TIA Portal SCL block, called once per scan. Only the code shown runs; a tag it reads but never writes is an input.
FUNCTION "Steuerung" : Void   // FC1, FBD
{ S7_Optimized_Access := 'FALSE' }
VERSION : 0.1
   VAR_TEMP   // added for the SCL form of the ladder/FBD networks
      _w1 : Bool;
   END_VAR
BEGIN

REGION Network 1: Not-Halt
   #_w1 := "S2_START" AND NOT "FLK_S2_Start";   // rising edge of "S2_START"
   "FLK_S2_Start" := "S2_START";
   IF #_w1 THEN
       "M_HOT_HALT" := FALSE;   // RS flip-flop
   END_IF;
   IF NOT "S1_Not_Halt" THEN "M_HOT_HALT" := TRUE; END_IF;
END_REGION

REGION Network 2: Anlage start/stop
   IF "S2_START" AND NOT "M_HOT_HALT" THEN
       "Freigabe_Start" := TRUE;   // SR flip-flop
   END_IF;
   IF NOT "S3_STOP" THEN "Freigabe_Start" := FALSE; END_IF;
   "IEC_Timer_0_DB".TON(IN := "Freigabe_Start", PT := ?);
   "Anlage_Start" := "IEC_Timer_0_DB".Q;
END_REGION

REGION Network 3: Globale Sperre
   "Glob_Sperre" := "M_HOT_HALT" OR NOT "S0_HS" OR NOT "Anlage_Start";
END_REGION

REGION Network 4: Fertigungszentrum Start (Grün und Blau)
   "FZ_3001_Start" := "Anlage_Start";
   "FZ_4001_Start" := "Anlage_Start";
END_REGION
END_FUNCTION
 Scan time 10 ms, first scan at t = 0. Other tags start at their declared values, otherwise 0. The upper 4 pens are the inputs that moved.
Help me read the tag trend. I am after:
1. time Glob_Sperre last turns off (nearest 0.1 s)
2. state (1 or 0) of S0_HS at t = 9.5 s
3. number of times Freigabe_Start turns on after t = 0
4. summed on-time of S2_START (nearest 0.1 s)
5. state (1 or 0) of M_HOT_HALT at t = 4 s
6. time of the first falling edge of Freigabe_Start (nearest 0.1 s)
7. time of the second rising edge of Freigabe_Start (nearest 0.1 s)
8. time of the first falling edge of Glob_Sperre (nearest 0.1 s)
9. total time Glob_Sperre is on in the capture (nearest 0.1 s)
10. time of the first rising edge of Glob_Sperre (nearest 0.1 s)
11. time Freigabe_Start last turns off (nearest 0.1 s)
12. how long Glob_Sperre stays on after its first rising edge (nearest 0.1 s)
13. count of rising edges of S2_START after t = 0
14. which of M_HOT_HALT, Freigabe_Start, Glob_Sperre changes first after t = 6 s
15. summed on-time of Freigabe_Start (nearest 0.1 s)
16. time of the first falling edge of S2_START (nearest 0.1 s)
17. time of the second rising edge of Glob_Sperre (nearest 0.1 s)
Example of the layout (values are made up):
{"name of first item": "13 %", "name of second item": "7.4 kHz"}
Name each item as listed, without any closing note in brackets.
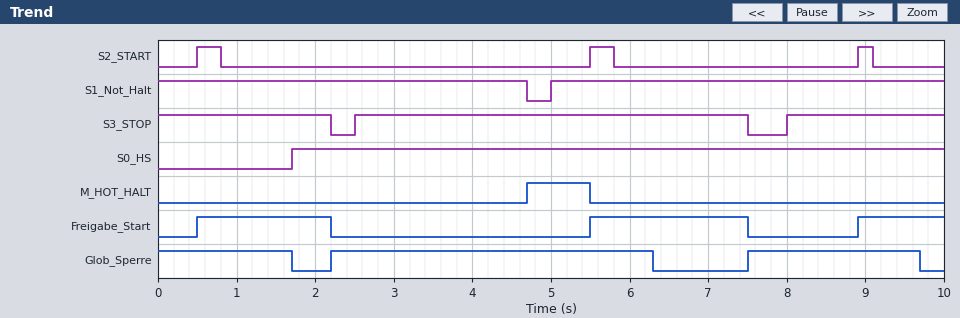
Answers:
{"time Glob_Sperre last turns off": "9.7 s", "state (1 or 0) of S0_HS at t = 9.5 s": "1", "number of times Freigabe_Start turns on after t = 0": "3", "summed on-time of S2_START": "0.8 s", "state (1 or 0) of M_HOT_HALT at t = 4 s": "0", "time of the first falling edge of Freigabe_Start": "2.2 s", "time of the second rising edge of Freigabe_Start": "5.5 s", "time of the first falling edge of Glob_Sperre": "1.7 s", "total time Glob_Sperre is on in the capture": "8.0 s", "time of the first rising edge of Glob_Sperre": "2.2 s", "time Freigabe_Start last turns off": "7.5 s", "how long Glob_Sperre stays on after its first rising edge": "4.1 s", "count of rising edges of S2_START after t = 0": "3", "which of M_HOT_HALT, Freigabe_Start, Glob_Sperre changes first after t = 6 s": "Glob_Sperre", "summed on-time of Freigabe_Start": "4.8 s", "time of the first falling edge of S2_START": "0.8 s", "time of the second rising edge of Glob_Sperre": "7.5 s"}
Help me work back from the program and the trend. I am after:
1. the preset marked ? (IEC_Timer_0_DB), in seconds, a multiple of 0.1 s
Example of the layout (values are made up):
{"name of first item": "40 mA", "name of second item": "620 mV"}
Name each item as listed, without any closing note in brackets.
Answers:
{"the preset marked ? (IEC_Timer_0_DB), in seconds, a multiple of 0.1 s": "0.8 s"}
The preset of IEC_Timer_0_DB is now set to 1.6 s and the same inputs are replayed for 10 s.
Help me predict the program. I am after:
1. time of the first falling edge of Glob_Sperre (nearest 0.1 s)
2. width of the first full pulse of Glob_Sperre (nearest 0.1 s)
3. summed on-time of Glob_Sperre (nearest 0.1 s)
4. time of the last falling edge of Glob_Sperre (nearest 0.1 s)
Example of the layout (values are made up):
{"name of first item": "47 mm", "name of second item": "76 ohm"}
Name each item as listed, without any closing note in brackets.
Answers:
{"time of the first falling edge of Glob_Sperre": "2.1 s", "width of the first full pulse of Glob_Sperre": "4.9 s", "summed on-time of Glob_Sperre": "9.5 s", "time of the last falling edge of Glob_Sperre": "7.1 s"}
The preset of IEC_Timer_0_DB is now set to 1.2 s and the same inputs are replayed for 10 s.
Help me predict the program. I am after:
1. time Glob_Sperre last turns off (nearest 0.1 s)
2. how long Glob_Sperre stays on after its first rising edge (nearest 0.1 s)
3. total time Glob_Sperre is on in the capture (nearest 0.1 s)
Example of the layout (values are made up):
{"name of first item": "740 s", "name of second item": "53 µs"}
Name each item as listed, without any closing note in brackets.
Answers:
{"time Glob_Sperre last turns off": "6.7 s", "how long Glob_Sperre stays on after its first rising edge": "4.5 s", "total time Glob_Sperre is on in the capture": "8.7 s"}
